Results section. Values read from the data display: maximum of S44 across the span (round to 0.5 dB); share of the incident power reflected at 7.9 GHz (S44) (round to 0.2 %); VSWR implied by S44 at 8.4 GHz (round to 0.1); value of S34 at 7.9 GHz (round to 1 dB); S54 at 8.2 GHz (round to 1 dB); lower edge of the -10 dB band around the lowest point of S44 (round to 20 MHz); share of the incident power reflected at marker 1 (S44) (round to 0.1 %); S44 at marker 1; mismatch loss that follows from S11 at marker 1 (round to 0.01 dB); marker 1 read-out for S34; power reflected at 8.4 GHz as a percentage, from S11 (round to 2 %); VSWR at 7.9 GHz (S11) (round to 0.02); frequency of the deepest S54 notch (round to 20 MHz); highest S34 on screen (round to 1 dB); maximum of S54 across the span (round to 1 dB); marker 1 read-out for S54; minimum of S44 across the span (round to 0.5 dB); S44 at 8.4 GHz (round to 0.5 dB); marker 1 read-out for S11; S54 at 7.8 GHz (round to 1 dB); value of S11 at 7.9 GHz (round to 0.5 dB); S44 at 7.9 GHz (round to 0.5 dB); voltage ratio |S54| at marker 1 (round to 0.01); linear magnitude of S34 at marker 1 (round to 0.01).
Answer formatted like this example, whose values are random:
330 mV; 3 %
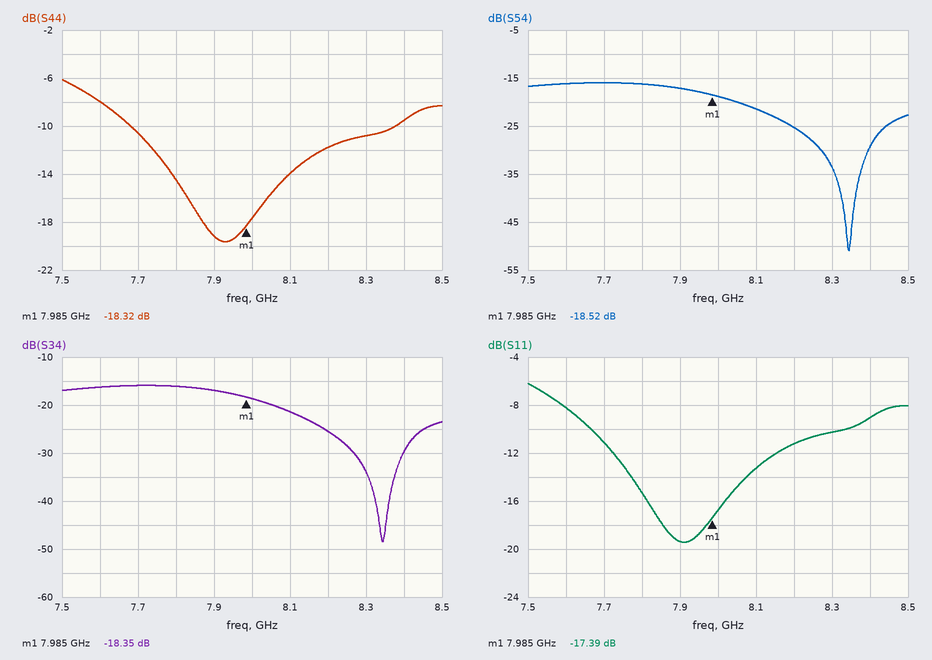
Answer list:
-6.0 dB; 1.2 %; 2.0; -17 dB; -25 dB; 7.68 GHz; 1.5 %; -18.32 dB; 0.08 dB; -18.35 dB; 12 %; 1.24; 8.34 GHz; -16 dB; -16 dB; -18.52 dB; -19.5 dB; -9.5 dB; -17.39 dB; -16 dB; -19.5 dB; -19.0 dB; 0.12; 0.12
